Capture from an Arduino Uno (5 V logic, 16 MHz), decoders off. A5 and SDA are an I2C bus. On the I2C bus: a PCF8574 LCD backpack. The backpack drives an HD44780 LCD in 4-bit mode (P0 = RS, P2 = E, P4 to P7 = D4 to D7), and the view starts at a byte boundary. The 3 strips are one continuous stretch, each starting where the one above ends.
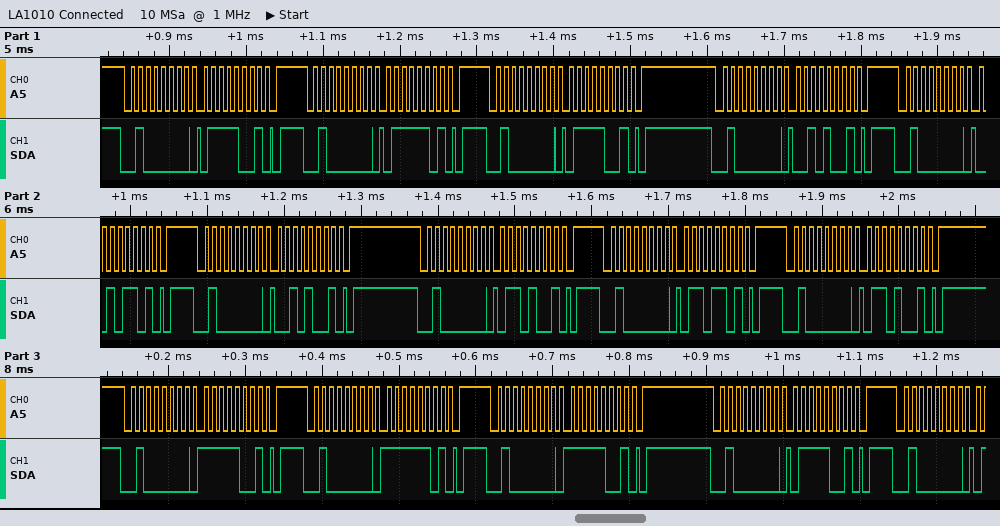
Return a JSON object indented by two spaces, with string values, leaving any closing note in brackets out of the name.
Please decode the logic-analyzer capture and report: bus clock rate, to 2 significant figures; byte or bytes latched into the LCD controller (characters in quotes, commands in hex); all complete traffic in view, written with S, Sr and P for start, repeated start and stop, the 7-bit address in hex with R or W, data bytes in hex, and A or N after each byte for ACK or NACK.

{
  "bus clock rate, to 2 significant figures": "100 kHz",
  "byte or bytes latched into the LCD controller": "'r' 'o'",
  "all complete traffic in view, written with S, Sr and P for start, repeated start and stop, the 7-bit address in hex with R or W, data bytes in hex, and A or N after each byte for ACK or NACK": "S 20W A 79 A P S 20W A 7D A P S 20W A 79 A P S 20W A 29 A P S 20W A 2D A P S 20W A 29 A P S 20W A 69 A P S 20W A 6D A P S 20W A 69 A P S 20W A F9 A P S 20W A FD A P S 20W A F9 A P S 20W A 79 A P S 20W A"
}
